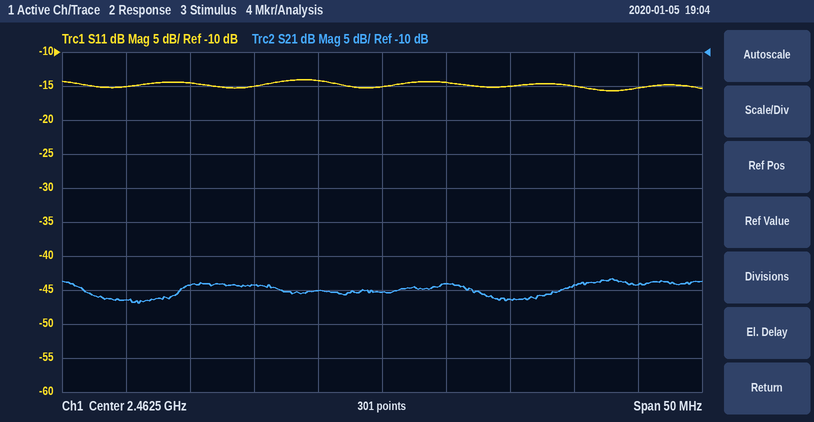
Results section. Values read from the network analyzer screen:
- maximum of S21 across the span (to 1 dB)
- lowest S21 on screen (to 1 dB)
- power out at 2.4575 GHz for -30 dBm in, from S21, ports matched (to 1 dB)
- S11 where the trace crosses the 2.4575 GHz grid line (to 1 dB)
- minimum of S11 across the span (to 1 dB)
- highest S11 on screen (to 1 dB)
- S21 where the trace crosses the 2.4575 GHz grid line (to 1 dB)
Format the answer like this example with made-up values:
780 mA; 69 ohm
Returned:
-43 dB; -47 dB; -75 dBm; -14 dB; -16 dB; -14 dB; -45 dB
